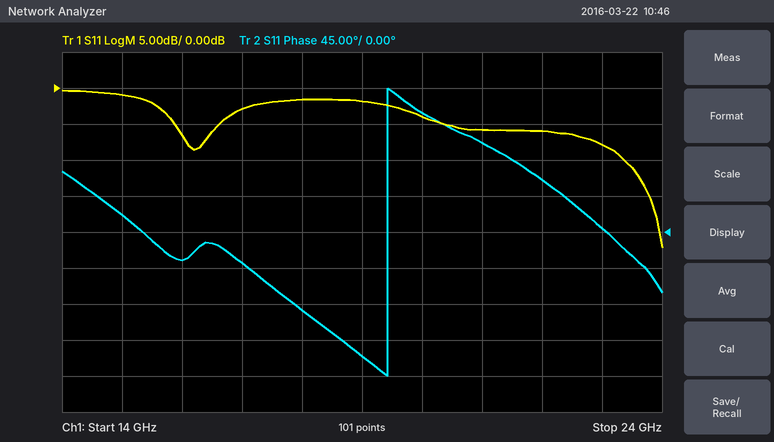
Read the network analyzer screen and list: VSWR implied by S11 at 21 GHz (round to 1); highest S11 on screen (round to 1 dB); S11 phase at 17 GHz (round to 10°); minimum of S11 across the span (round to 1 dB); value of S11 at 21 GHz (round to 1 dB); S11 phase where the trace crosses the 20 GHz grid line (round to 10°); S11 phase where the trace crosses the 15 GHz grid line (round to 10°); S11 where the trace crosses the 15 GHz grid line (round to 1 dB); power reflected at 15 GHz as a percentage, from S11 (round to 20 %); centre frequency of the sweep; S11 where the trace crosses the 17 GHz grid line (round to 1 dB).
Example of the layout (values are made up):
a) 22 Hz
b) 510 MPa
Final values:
a) 3
b) 0 dB
c) -40°
d) -22 dB
e) -6 dB
f) 150°
g) 20°
h) -1 dB
i) 80 %
j) 19 GHz
k) -3 dB
